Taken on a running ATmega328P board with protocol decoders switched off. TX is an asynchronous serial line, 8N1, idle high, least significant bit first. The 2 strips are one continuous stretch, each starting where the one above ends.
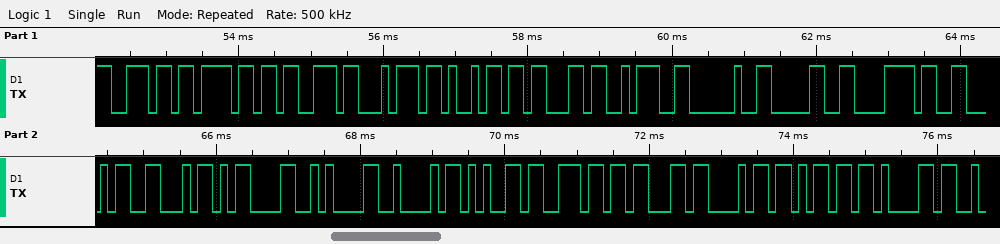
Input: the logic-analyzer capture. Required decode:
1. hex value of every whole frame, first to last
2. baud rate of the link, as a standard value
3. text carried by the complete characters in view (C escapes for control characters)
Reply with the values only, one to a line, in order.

0x6E 0x6F 0x73 0x74 0x69 0x63 0x3A 0x20 0x30 0x78 0x46 0x46 0x0D 0x0A 0x42 0x65 0x6E 0x63 0x68 0x6D 0x61
9600 baud
"nostic: 0xFF\r\nBenchma"
